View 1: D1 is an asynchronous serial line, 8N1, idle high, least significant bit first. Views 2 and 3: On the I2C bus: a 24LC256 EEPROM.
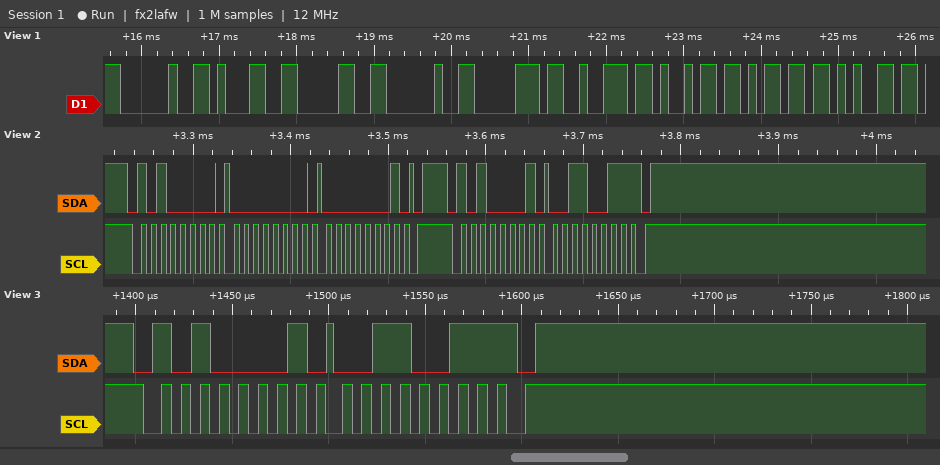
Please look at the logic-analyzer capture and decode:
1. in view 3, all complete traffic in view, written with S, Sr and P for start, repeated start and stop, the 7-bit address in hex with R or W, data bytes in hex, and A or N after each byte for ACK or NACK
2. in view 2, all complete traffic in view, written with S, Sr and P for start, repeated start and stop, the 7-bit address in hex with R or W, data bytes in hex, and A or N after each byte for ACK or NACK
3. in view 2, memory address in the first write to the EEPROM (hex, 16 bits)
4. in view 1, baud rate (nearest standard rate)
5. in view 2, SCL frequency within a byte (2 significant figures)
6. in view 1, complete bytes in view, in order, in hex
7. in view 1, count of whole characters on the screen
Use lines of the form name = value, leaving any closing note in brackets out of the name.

in view 3, all complete traffic in view, written with S, Sr and P for start, repeated start and stop, the 7-bit address in hex with R or W, data bytes in hex, and A or N after each byte for ACK or NACK = S 50R A 33 N P
in view 2, all complete traffic in view, written with S, Sr and P for start, repeated start and stop, the 7-bit address in hex with R or W, data bytes in hex, and A or N after each byte for ACK or NACK = S 50W A 00 A 01 A P S 50R A 33 N P
in view 2, memory address in the first write to the EEPROM = 0x0001
in view 1, baud rate = 9600 baud
in view 2, SCL frequency within a byte = 100 kHz
in view 1, complete bytes in view, in order, in hex = 20 31 30 20 70 72 69 6D 65
in view 1, count of whole characters on the screen = 9
